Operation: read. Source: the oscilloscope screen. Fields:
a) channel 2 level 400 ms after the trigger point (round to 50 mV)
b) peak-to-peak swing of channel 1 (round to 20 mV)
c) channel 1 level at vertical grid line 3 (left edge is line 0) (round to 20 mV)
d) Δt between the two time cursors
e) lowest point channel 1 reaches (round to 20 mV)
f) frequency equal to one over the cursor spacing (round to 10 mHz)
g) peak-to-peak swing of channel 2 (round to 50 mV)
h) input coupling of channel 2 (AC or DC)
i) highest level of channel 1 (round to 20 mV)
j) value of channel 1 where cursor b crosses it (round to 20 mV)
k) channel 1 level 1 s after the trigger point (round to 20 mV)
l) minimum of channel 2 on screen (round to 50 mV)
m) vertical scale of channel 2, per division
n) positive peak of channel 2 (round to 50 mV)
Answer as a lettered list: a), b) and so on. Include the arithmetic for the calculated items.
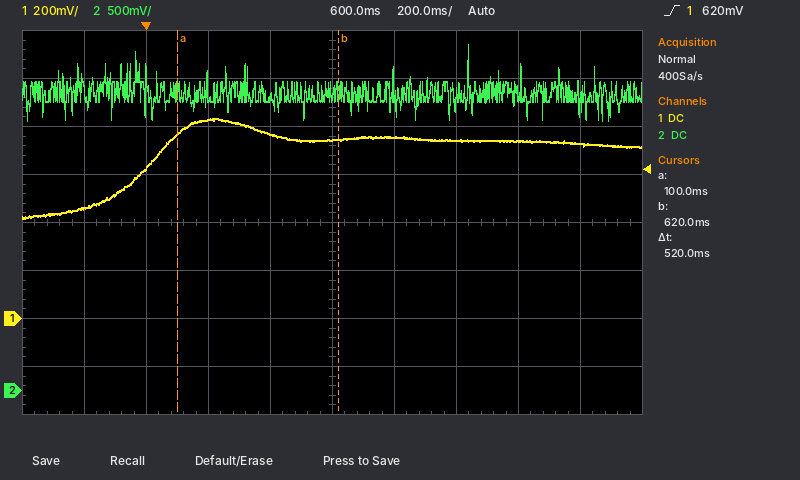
a) 3.05 V
b) 840 mV − (420 mV) = 420 mV
c) 820 mV
d) 520 ms
e) 420 mV
f) 1 / 520 ms ≈ 1.92 Hz
g) 3.60 V − (2.80 V) = 800 mV
h) DC
i) 840 mV
j) 740 mV
k) 740 mV
l) 2.80 V
m) 500 mV
n) 3.60 V
